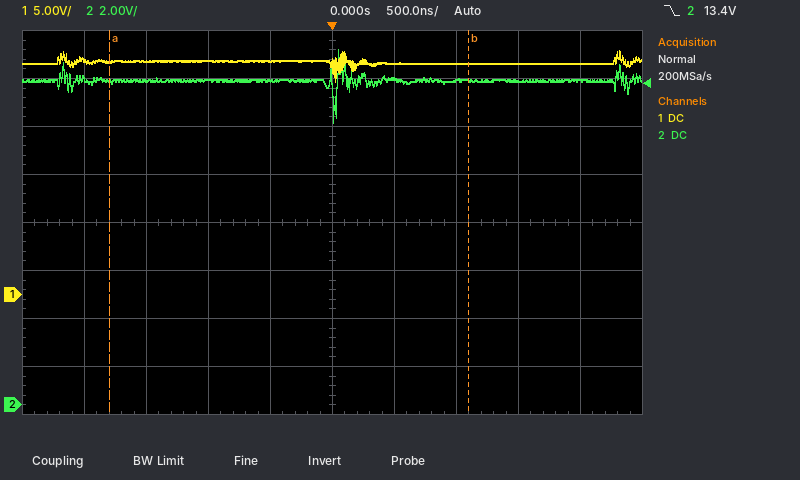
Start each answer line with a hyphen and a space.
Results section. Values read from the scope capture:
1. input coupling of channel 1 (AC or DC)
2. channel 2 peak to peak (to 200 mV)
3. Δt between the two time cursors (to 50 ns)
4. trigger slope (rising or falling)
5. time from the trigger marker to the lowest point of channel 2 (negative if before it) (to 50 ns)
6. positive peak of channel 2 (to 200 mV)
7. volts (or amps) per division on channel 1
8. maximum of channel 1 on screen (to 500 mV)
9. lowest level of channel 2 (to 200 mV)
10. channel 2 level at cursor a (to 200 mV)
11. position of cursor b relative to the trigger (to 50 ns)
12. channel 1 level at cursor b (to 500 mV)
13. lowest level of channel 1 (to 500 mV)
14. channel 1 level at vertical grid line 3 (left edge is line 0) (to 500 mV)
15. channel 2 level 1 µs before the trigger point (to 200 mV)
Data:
- DC
- 3.0 V
- 2.90 µs
- falling
- 0 ns
- 14.8 V
- 5 V
- 25.5 V
- 11.8 V
- 13.4 V
- +1.10 µs
- 24.0 V
- 22.0 V
- 24.5 V
- 13.6 V
